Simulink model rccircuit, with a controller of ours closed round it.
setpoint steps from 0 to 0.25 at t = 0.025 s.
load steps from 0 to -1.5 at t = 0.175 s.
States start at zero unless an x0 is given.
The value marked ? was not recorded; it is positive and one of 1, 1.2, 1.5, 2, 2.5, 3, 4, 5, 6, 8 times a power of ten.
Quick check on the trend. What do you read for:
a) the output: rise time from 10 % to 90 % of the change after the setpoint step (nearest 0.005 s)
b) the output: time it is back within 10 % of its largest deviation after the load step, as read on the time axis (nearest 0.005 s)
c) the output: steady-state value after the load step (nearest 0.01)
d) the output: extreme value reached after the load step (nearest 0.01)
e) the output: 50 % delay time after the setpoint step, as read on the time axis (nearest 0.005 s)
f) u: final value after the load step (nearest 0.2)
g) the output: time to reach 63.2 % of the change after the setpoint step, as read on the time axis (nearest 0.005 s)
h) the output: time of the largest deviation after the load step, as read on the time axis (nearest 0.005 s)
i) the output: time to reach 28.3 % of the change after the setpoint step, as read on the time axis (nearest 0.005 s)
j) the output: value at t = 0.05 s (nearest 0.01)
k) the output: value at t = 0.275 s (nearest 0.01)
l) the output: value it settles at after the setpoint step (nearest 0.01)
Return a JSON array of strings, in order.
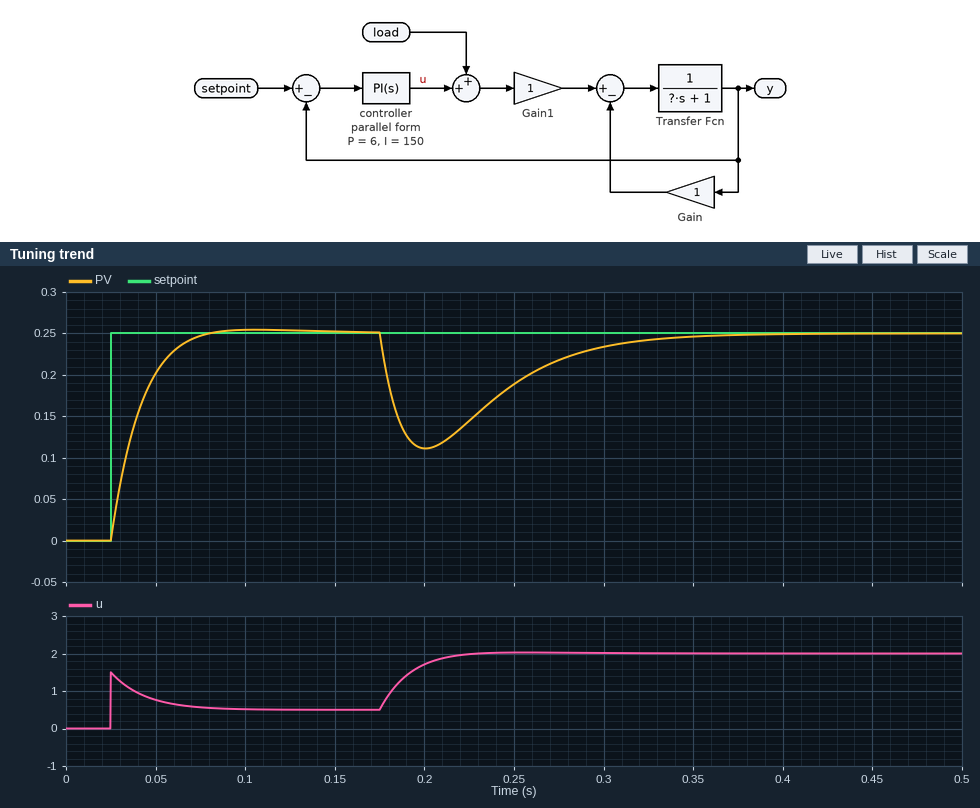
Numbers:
["0.030 s", "0.305 s", "0.25", "0.11", "0.035 s", "2.0", "0.040 s", "0.200 s", "0.030 s", "0.20", "0.22", "0.25"]
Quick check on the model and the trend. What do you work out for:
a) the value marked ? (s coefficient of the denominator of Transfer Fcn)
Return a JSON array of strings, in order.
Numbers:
["0.1"]
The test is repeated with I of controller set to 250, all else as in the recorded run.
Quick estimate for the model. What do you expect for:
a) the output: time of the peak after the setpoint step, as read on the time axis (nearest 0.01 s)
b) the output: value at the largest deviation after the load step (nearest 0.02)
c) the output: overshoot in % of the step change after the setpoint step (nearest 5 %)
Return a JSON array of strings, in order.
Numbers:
["0.08 s", "0.12", "10 %"]
